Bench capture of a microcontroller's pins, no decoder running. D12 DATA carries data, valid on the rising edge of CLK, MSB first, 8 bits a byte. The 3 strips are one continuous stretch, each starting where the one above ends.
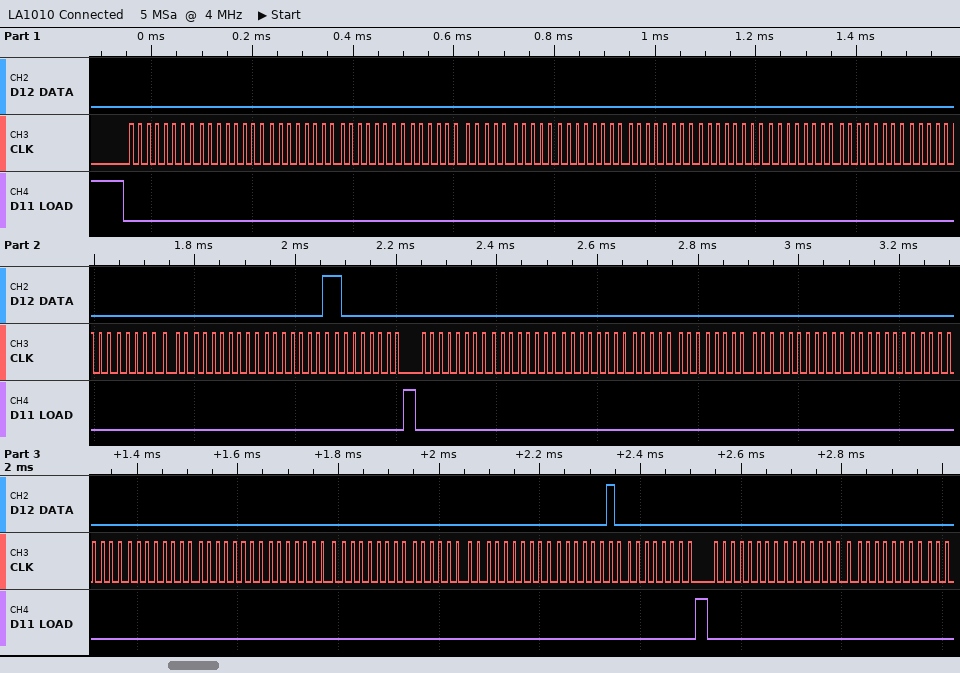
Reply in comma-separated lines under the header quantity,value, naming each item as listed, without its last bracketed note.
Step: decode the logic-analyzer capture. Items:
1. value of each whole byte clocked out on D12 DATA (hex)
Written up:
quantity,value
value of each whole byte clocked out on D12 DATA,00 00 00 00 00 00 00 00 00 00 00 00 00 00 01 80 00 00 00 00 00 00 00 00 00 00 00 00 00 00 02 00 00 00 00
